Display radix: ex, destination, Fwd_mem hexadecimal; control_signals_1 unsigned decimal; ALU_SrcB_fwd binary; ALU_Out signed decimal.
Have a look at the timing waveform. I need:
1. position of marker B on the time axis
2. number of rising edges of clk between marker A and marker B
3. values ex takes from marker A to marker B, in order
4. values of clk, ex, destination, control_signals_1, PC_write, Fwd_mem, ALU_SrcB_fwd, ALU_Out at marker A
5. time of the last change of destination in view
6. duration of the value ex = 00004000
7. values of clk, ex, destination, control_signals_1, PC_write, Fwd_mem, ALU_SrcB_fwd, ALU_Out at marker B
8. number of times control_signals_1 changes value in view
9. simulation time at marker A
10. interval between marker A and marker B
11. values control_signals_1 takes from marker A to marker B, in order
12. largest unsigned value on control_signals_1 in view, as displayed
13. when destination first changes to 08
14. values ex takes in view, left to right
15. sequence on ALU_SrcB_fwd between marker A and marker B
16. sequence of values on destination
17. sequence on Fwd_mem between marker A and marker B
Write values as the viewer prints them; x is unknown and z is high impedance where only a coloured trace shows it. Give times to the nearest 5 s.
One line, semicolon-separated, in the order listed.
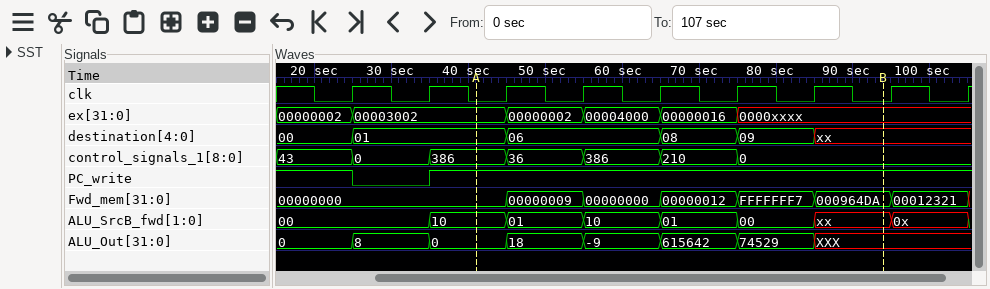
95 s; 5; 00003002, 00000002, 00004000, 00000016, 0000xxxx; clk=0, ex=00003002, destination=01, control_signals_1=386, PC_write=1, Fwd_mem=00000000, ALU_SrcB_fwd=10, ALU_Out=0; 85 s; 10 s; clk=0, ex=0000xxxx, destination=xx, control_signals_1=0, PC_write=1, Fwd_mem=000964DA, ALU_SrcB_fwd=xx, ALU_Out=XXX; 6; 40 s; 55 s; 386, 36, 386, 210, 0; 386; 65 s; 00000002, 00003002, 00000002, 00004000, 00000016, 0000xxxx; 10, 01, 10, 01, 00, xx; 00, 01, 06, 08, 09, xx; 00000000, 00000009, 00000000, 00000012, FFFFFFF7, 000964DA
